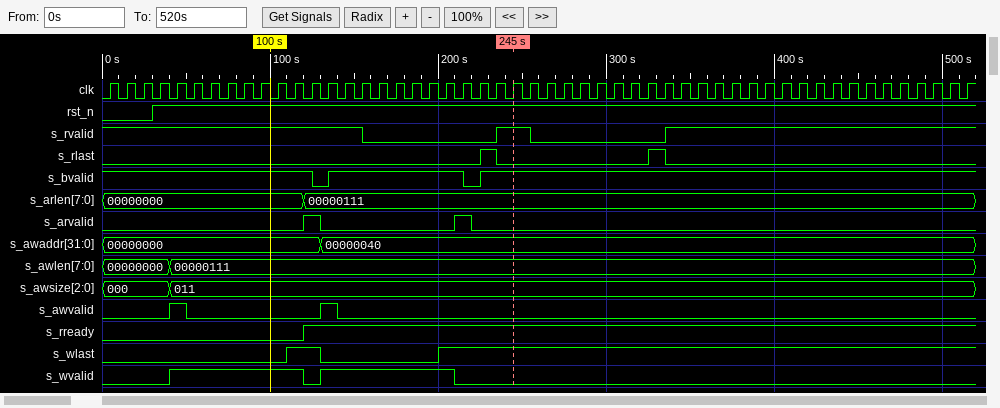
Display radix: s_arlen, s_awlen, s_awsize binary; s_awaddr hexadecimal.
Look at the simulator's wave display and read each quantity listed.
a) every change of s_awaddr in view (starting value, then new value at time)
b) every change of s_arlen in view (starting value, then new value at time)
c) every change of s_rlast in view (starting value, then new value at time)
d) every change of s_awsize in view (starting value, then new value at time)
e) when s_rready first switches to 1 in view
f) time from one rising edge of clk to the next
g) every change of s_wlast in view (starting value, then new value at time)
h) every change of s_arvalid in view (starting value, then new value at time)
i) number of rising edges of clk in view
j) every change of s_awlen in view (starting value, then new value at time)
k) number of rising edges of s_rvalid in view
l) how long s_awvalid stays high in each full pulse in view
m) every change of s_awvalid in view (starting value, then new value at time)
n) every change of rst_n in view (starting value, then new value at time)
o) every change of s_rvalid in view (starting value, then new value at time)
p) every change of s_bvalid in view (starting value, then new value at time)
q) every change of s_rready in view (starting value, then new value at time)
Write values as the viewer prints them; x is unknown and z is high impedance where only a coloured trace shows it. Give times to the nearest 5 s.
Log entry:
00000000, 00000040 at 130 s
00000000, 00000111 at 120 s
0, 1 at 225 s, 0 at 235 s, 1 at 325 s, 0 at 335 s
000, 011 at 40 s
120 s
10 s
0, 1 at 110 s, 0 at 130 s, 1 at 200 s
0, 1 at 120 s, 0 at 130 s, 1 at 210 s, 0 at 220 s
52
00000000, 00000111 at 40 s
2
10 s, 10 s
0, 1 at 40 s, 0 at 50 s, 1 at 130 s, 0 at 140 s
0, 1 at 30 s
1, 0 at 155 s, 1 at 235 s, 0 at 255 s, 1 at 335 s
1, 0 at 125 s, 1 at 135 s, 0 at 215 s, 1 at 225 s
0, 1 at 120 s
